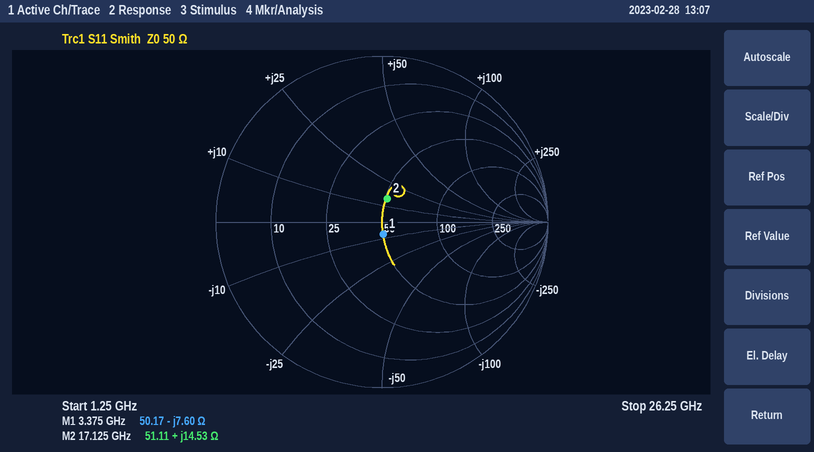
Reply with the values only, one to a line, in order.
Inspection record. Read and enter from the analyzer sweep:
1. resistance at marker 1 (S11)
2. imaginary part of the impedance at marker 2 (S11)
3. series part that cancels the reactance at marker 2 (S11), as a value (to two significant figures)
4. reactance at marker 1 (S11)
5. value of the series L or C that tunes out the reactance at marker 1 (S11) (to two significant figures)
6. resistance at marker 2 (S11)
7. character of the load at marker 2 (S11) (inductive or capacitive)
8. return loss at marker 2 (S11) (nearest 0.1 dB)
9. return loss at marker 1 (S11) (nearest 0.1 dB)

50.17 Ω
+14.53 Ω
640 fF
-7.60 Ω
360 pH
51.11 Ω
inductive
16.9 dB
22.4 dB
